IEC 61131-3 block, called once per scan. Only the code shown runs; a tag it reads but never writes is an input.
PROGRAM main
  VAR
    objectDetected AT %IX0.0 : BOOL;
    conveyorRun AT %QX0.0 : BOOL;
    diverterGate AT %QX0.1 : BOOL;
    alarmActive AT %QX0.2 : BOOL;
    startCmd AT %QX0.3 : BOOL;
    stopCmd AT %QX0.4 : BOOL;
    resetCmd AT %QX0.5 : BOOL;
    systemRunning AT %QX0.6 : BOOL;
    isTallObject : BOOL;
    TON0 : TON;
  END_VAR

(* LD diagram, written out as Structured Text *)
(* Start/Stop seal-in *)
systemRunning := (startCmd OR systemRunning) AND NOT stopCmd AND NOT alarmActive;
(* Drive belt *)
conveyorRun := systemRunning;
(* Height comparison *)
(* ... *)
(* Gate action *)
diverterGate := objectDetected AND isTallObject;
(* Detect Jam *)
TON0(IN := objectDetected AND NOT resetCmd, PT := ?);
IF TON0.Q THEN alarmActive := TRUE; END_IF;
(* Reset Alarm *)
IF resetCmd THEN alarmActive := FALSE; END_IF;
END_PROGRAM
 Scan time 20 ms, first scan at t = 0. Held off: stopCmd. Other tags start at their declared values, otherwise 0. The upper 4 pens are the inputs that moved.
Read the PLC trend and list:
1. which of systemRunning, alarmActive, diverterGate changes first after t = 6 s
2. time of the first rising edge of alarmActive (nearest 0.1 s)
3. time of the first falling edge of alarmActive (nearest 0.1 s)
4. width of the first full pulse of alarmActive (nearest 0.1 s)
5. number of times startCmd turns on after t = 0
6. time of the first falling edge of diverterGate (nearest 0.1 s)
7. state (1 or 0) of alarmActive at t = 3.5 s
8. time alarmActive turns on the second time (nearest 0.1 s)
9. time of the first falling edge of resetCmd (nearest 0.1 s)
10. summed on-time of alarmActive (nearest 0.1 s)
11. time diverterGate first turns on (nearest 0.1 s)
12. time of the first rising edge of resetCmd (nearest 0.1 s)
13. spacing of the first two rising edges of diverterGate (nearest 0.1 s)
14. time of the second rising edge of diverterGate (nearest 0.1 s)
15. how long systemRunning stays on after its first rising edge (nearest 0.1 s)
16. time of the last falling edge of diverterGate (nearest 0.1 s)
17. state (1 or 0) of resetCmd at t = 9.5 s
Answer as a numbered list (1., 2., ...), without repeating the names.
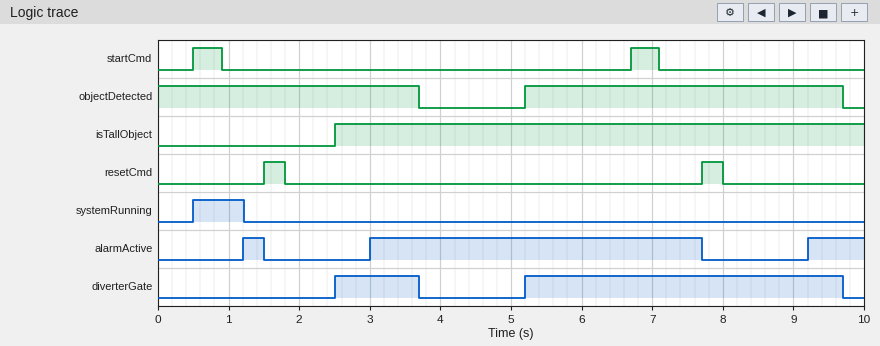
1. alarmActive
2. 1.2 s
3. 1.5 s
4. 0.3 s
5. 2
6. 3.7 s
7. 1
8. 3.0 s
9. 1.8 s
10. 5.8 s
11. 2.5 s
12. 1.5 s
13. 2.7 s
14. 5.2 s
15. 0.7 s
16. 9.7 s
17. 0
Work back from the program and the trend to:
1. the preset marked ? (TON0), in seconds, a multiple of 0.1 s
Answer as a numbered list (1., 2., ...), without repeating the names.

1. 1.2 s
